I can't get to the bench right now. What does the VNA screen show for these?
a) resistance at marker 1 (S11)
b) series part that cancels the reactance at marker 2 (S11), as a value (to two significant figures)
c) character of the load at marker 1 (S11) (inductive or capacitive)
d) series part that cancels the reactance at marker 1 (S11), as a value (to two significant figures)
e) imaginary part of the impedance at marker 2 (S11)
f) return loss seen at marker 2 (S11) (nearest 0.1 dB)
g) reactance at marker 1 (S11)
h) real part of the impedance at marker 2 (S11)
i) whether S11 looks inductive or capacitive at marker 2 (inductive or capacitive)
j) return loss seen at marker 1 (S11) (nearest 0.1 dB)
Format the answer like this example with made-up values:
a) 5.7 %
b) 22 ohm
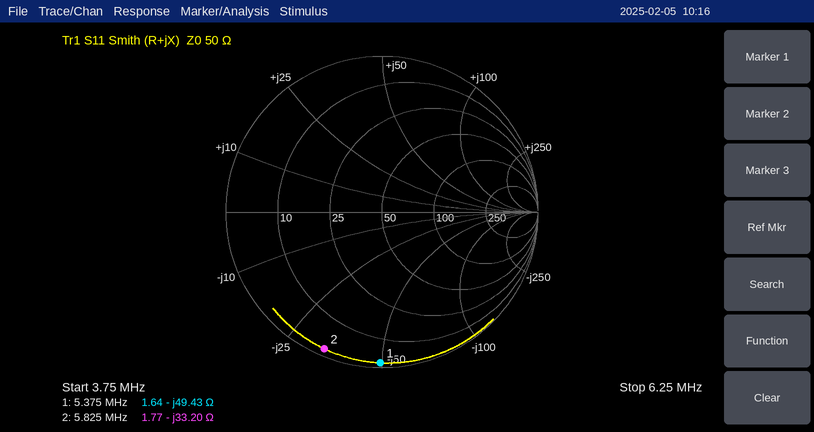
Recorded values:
a) 1.64 Ω
b) 910 nH
c) capacitive
d) 1.5 µH
e) -33.20 Ω
f) 0.4 dB
g) -49.43 Ω
h) 1.77 Ω
i) capacitive
j) 0.3 dB
